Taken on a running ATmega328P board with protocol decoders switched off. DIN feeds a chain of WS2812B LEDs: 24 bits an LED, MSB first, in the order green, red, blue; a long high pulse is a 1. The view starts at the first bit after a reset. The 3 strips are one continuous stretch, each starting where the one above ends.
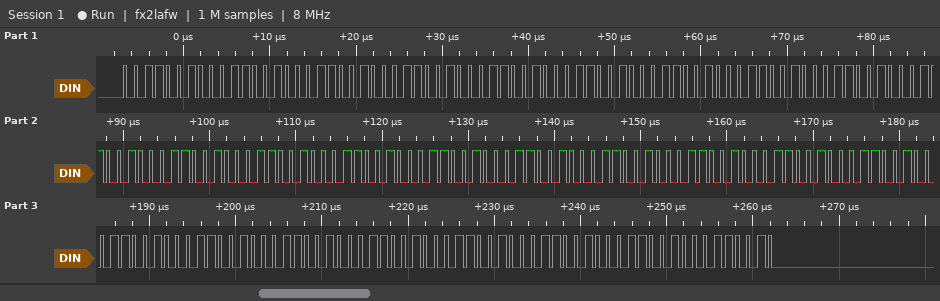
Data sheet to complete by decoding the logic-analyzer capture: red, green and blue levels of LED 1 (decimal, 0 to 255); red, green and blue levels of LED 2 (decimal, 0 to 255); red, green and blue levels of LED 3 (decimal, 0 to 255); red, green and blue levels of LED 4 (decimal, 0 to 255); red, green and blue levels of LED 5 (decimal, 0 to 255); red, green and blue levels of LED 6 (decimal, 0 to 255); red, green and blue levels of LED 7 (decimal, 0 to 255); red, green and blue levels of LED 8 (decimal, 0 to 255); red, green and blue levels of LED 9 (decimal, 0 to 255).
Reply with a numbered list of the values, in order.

1. 50, 50, 50
2. 50, 50, 50
3. 50, 50, 50
4. 50, 50, 50
5. 50, 50, 50
6. 50, 50, 50
7. 50, 50, 50
8. 50, 50, 50
9. 50, 50, 50
